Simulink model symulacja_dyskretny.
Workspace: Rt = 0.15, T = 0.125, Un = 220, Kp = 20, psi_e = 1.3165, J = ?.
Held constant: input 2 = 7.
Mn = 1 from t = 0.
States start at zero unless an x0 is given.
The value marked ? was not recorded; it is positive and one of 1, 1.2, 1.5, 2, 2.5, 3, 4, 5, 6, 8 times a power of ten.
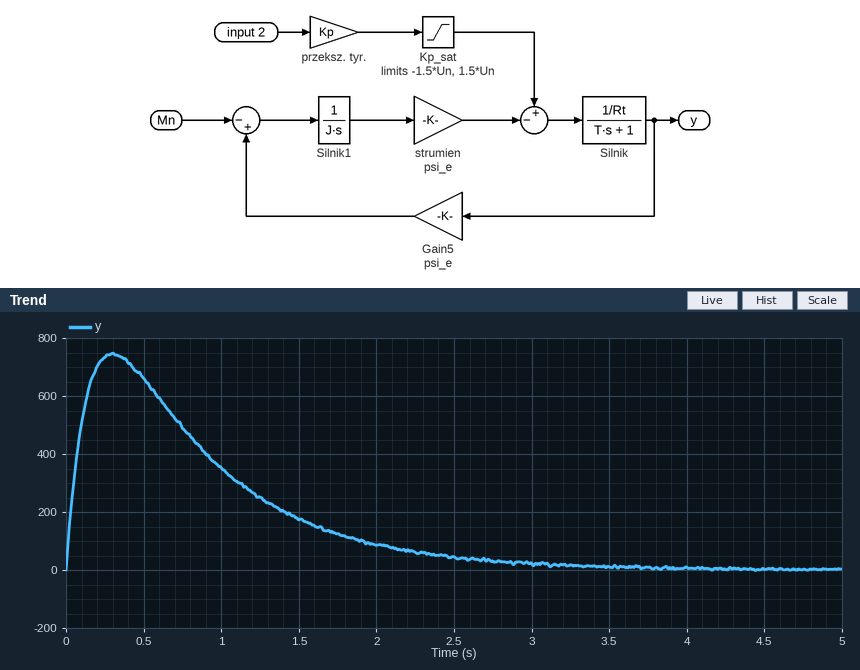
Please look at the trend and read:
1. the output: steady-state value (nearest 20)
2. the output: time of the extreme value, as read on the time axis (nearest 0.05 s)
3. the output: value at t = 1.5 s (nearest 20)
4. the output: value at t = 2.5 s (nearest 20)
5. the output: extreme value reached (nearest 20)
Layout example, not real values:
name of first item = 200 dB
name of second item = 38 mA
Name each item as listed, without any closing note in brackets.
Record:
the output: steady-state value = 0
the output: time of the extreme value, as read on the time axis = 0.30 s
the output: value at t = 1.5 s = 180
the output: value at t = 2.5 s = 40
the output: extreme value reached = 740
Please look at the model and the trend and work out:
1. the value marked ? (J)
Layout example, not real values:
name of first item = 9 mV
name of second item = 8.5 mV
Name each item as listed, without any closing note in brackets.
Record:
the value marked ? = 10
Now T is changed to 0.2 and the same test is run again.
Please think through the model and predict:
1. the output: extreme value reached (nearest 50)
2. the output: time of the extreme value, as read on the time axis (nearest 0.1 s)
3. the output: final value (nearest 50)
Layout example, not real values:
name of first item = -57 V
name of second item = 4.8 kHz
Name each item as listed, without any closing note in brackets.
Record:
the output: extreme value reached = 700
the output: time of the extreme value, as read on the time axis = 0.4 s
the output: final value = 0
